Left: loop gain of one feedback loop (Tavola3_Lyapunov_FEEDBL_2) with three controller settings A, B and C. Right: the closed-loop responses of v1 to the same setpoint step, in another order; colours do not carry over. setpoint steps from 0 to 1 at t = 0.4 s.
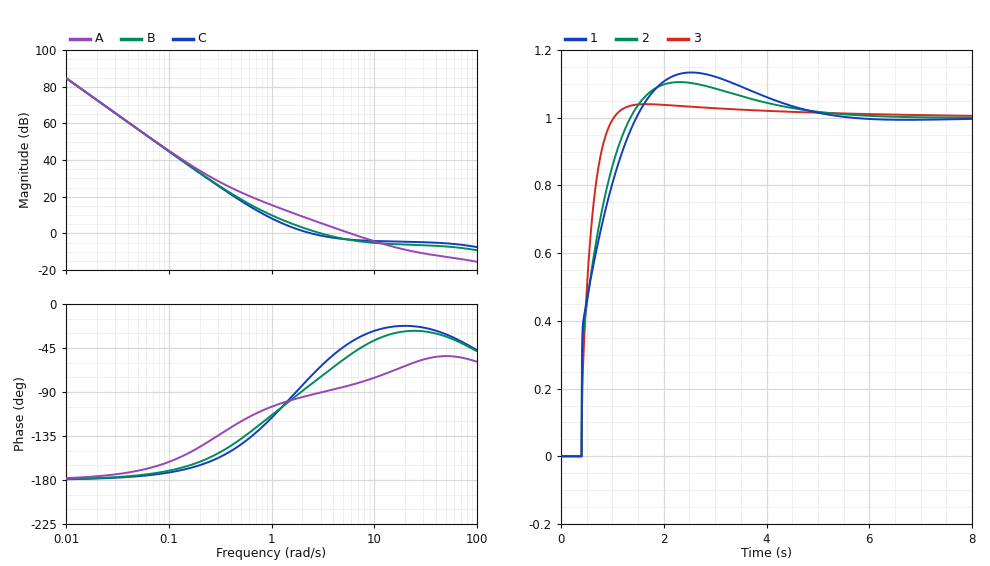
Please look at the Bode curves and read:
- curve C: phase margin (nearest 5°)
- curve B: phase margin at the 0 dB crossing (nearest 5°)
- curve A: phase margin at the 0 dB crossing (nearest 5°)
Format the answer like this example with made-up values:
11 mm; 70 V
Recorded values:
105°; 105°; 95°
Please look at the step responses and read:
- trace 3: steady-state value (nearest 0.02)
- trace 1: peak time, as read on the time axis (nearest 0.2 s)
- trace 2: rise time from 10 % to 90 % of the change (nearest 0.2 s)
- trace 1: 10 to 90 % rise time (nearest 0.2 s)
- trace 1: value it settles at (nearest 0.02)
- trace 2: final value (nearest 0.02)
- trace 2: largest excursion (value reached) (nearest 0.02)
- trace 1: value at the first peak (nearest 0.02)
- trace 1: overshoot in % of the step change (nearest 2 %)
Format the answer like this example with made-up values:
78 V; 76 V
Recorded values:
1.00; 2.6 s; 0.6 s; 0.8 s; 1.00; 1.00; 1.10; 1.14; 14 %
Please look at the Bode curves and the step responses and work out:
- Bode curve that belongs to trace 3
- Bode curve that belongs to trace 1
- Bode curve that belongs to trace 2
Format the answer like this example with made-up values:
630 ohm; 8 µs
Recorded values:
A; C; B
